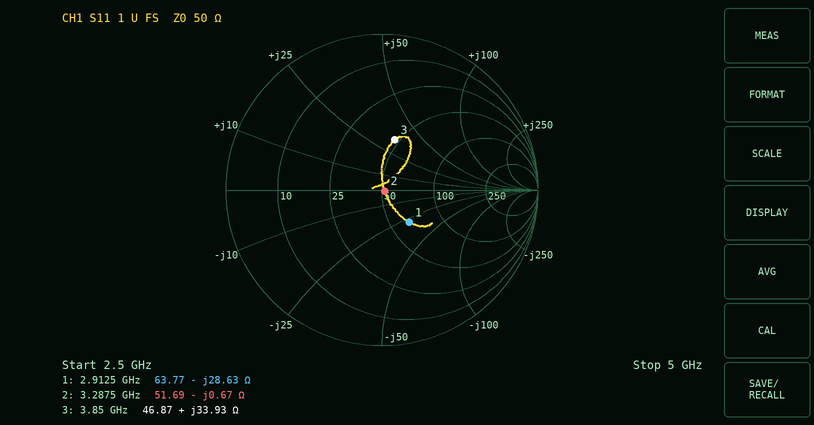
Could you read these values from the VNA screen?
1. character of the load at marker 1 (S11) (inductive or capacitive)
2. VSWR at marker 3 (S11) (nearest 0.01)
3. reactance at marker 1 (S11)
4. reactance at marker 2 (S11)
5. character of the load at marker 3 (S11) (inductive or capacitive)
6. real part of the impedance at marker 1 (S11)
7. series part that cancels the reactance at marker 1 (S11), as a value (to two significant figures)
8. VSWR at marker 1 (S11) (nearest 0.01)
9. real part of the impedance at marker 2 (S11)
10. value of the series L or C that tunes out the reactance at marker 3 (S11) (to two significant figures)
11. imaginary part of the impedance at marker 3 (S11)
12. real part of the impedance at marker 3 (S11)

capacitive
1.99
-28.63 Ω
-0.67 Ω
inductive
63.77 Ω
1.6 nH
1.74
51.69 Ω
1.2 pF
+33.93 Ω
46.87 Ω
